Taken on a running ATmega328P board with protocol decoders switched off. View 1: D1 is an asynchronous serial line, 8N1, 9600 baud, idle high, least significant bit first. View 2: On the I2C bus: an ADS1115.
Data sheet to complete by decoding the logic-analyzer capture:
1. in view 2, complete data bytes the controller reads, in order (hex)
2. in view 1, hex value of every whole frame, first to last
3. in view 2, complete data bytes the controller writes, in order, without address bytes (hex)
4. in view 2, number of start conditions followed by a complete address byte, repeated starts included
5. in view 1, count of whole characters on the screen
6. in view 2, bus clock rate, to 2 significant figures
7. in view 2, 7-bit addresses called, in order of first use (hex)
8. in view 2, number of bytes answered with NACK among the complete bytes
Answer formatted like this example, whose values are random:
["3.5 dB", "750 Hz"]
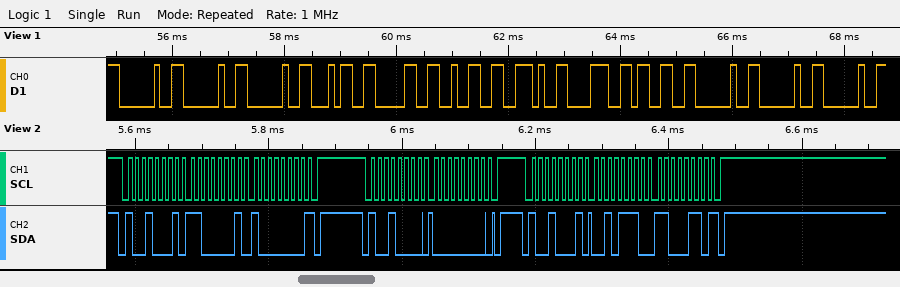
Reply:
["C1 80 2E C6", "20 20 20 34 30 32 2E 38 33 20 20 20", "00", "3", "12", "100 kHz", "0x48", "2"]
